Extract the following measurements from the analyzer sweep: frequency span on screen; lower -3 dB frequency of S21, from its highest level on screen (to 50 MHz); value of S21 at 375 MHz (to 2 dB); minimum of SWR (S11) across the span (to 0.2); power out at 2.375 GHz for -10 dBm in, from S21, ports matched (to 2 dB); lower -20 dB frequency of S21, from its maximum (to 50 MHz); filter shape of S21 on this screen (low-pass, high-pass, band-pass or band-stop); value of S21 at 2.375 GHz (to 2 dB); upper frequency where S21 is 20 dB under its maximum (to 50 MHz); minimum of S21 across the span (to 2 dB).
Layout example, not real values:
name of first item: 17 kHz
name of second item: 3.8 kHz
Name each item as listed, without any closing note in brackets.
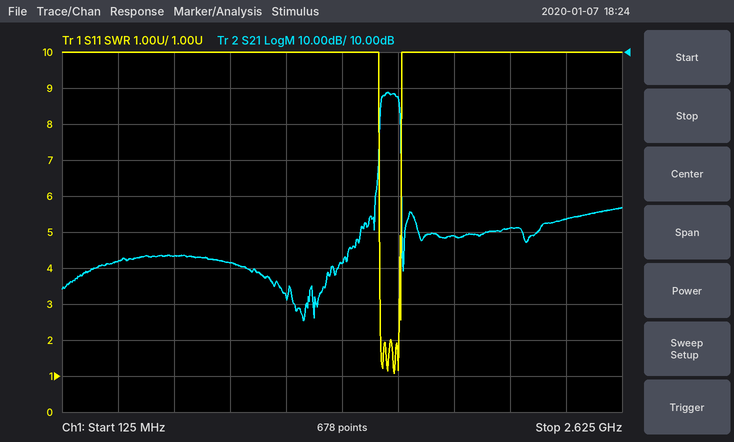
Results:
frequency span on screen: 2.5 GHz
lower -3 dB frequency of S21, from its highest level on screen: 1.55 GHz
value of S21 at 375 MHz: -48 dB
minimum of SWR (S11) across the span: 1.0
power out at 2.375 GHz for -10 dBm in, from S21, ports matched: -46 dBm
lower -20 dB frequency of S21, from its maximum: 1.55 GHz
filter shape of S21 on this screen: band-pass
value of S21 at 2.375 GHz: -36 dB
upper frequency where S21 is 20 dB under its maximum: 1.65 GHz
minimum of S21 across the span: -64 dB
